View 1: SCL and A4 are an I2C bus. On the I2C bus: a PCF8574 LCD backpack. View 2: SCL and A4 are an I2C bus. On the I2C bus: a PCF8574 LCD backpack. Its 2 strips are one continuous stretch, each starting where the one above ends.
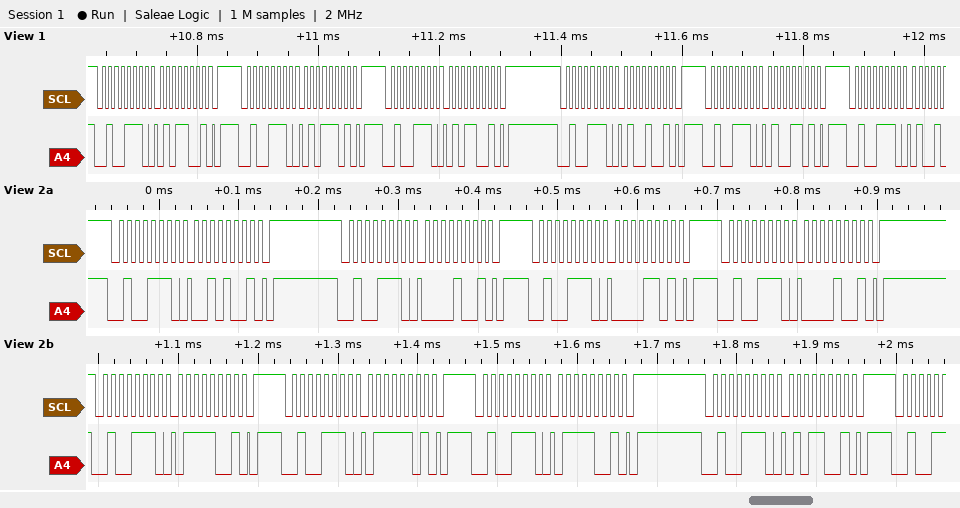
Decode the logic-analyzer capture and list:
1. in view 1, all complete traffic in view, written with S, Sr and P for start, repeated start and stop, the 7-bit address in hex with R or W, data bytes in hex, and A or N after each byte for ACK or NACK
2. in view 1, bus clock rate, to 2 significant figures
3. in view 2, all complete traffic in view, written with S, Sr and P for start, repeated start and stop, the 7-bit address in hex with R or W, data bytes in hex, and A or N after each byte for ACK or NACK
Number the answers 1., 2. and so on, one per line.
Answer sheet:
1. S 27W A 59 A P S 27W A 5D A P S 27W A 59 A P S 27W A 49 A P S 27W A 4D A P S 27W A
2. 100 kHz
3. S 27W A 29 A P S 27W A 09 A P S 27W A 0D A P S 27W A 09 A P S 27W A 79 A P S 27W A 7D A P S 27W A 79 A P S 27W A 59 A P
